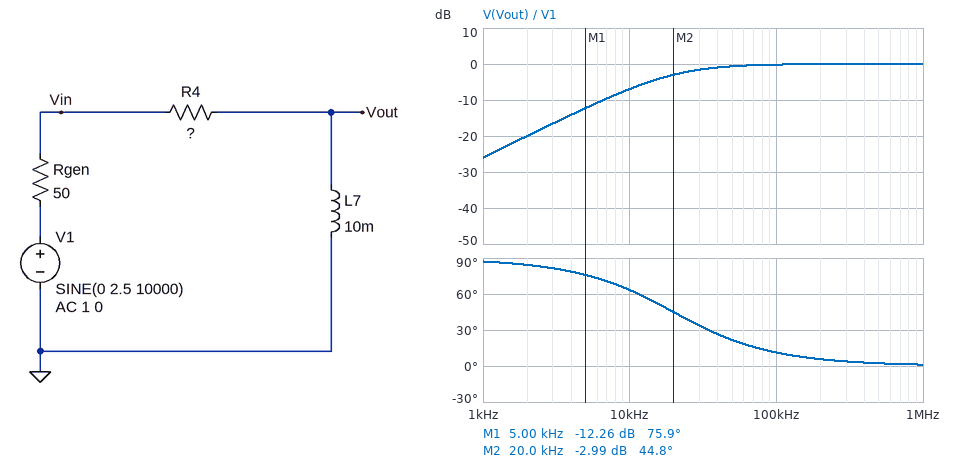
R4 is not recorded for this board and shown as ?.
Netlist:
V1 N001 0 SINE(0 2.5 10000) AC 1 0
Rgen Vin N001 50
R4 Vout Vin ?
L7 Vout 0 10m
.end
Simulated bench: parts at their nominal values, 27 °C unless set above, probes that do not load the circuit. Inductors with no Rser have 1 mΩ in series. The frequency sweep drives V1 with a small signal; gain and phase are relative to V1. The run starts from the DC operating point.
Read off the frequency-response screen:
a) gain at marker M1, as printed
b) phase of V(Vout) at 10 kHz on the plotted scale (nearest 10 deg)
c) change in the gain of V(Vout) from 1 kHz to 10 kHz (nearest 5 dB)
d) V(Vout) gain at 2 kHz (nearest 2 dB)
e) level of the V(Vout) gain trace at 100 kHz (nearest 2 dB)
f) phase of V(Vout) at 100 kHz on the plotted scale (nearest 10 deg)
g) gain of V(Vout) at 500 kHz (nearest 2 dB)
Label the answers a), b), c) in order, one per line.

a) -12.26 dB
b) 60 deg
c) 20 dB
d) -20 dB
e) 0 dB
f) 10 deg
g) 0 dB
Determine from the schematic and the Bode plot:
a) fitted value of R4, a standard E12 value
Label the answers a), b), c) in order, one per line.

a) 1.2 kΩ
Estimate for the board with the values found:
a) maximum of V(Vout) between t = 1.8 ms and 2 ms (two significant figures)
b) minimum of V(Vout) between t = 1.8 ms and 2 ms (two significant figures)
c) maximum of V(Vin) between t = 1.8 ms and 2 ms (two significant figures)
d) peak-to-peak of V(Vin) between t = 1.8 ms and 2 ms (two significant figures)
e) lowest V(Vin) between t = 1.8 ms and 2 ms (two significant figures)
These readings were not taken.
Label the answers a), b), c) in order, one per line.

a) 1.1 V
b) -1.1 V
c) 2.4 V
d) 4.8 V
e) -2.4 V
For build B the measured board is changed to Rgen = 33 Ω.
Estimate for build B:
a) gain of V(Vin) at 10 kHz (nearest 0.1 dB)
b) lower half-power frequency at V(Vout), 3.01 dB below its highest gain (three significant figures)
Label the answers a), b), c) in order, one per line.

a) -0.2 dB
b) 19.6 kHz
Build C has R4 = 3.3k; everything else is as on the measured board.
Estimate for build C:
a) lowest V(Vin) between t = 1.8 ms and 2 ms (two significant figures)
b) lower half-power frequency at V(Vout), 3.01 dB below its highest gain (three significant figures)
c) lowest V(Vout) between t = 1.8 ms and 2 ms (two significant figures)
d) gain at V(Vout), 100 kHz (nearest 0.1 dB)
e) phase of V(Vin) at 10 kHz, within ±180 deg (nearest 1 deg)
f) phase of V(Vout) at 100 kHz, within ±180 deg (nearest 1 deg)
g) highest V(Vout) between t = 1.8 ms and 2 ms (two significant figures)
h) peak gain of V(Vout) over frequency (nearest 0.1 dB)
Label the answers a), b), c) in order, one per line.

a) -2.5 V
b) 53.3 kHz
c) -460 mV
d) -1.1 dB
e) 0 deg
f) 28 deg
g) 460 mV
h) 0 dB
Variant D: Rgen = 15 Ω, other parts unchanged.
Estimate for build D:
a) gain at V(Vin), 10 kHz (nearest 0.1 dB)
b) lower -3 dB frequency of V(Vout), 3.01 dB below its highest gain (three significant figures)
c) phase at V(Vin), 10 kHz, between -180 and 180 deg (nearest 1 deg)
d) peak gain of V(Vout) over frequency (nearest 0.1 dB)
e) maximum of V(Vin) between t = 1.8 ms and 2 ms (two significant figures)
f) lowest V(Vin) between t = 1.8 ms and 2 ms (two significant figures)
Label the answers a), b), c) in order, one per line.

a) -0.1 dB
b) 19.3 kHz
c) 0 deg
d) 0 dB
e) 2.5 V
f) -2.5 V
